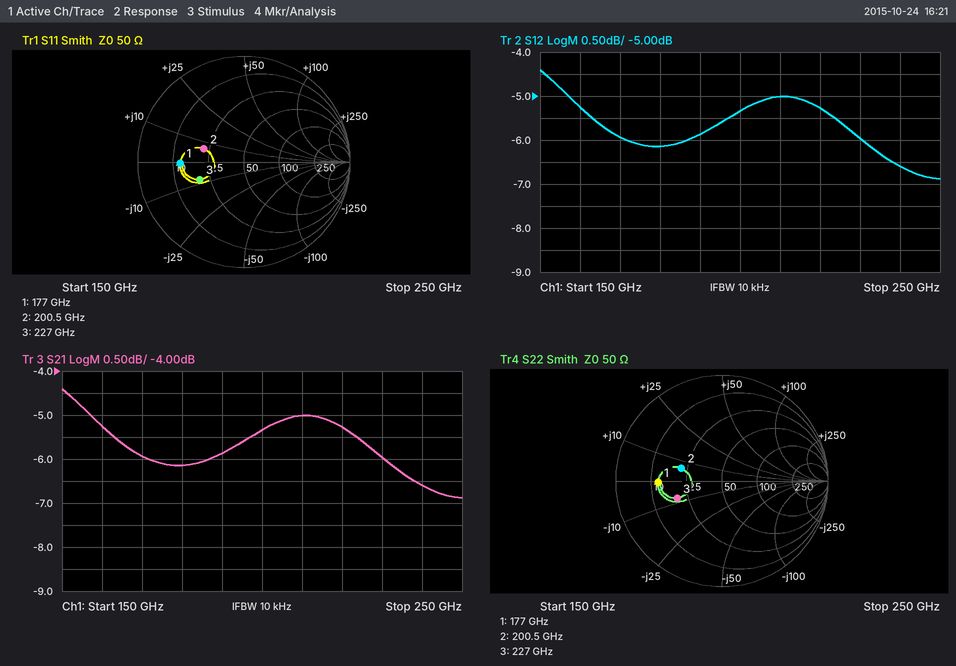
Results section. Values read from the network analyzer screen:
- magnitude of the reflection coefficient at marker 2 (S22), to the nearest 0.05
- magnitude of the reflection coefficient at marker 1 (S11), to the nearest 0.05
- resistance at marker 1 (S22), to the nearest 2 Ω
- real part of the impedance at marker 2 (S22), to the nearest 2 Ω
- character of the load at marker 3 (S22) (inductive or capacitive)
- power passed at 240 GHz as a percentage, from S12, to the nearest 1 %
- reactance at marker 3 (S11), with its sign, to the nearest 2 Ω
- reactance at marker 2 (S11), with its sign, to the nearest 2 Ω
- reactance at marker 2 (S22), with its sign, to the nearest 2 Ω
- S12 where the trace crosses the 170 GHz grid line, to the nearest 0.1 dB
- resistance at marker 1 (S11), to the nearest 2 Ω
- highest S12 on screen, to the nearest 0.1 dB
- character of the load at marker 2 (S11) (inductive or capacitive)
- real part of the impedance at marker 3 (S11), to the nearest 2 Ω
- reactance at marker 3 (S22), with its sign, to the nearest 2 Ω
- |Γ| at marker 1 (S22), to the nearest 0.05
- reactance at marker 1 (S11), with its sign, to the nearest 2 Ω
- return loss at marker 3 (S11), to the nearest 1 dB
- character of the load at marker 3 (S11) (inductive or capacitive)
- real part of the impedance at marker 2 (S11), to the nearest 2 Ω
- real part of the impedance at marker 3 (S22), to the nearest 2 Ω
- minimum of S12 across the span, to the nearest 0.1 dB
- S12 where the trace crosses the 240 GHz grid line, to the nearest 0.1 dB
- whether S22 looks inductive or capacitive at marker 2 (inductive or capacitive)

0.40
0.60
12 Ω
22 Ω
capacitive
22 %
-8 Ω
+6 Ω
+6 Ω
-5.9 dB
12 Ω
-4.4 dB
inductive
20 Ω
-8 Ω
0.60
0 Ω
7 dB
capacitive
22 Ω
20 Ω
-6.9 dB
-6.6 dB
inductive
